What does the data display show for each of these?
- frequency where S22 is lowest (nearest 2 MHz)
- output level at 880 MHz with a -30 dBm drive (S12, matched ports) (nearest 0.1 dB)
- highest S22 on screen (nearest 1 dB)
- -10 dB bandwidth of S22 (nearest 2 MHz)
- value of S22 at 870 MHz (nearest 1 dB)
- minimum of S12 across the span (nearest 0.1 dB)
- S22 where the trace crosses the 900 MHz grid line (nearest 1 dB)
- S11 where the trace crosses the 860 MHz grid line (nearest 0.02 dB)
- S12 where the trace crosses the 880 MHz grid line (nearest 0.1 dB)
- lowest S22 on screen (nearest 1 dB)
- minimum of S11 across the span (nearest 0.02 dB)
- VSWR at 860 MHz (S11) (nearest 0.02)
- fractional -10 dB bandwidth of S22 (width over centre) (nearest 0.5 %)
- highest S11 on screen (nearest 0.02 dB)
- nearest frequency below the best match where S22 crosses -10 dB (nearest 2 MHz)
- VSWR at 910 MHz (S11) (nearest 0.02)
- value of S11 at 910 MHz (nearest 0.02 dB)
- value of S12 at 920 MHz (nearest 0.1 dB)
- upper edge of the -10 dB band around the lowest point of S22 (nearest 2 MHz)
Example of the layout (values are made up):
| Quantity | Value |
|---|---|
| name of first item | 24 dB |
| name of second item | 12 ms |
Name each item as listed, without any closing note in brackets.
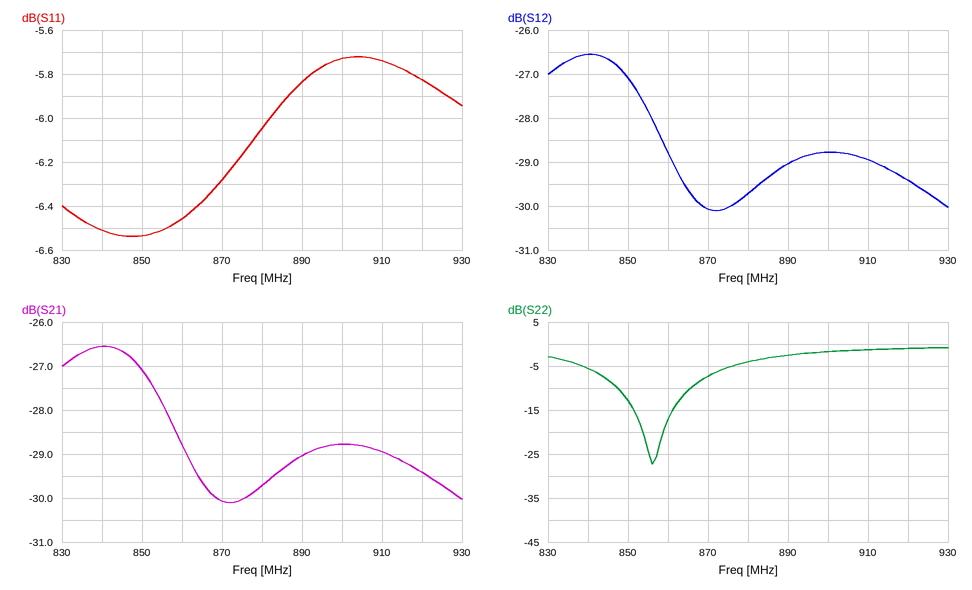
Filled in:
| Quantity | Value |
|---|---|
| frequency where S22 is lowest | 856 MHz |
| output level at 880 MHz with a -30 dBm drive (S12, matched ports) | -59.7 dBm |
| highest S22 on screen | -1 dB |
| -10 dB bandwidth of S22 | 18 MHz |
| value of S22 at 870 MHz | -7 dB |
| minimum of S12 across the span | -30.1 dB |
| S22 where the trace crosses the 900 MHz grid line | -2 dB |
| S11 where the trace crosses the 860 MHz grid line | -6.46 dB |
| S12 where the trace crosses the 880 MHz grid line | -29.7 dB |
| lowest S22 on screen | -27 dB |
| minimum of S11 across the span | -6.54 dB |
| VSWR at 860 MHz (S11) | 2.82 |
| fractional -10 dB bandwidth of S22 (width over centre) | 2.0 % |
| highest S11 on screen | -5.72 dB |
| nearest frequency below the best match where S22 crosses -10 dB | 848 MHz |
| VSWR at 910 MHz (S11) | 3.14 |
| value of S11 at 910 MHz | -5.74 dB |
| value of S12 at 920 MHz | -29.4 dB |
| upper edge of the -10 dB band around the lowest point of S22 | 866 MHz |
